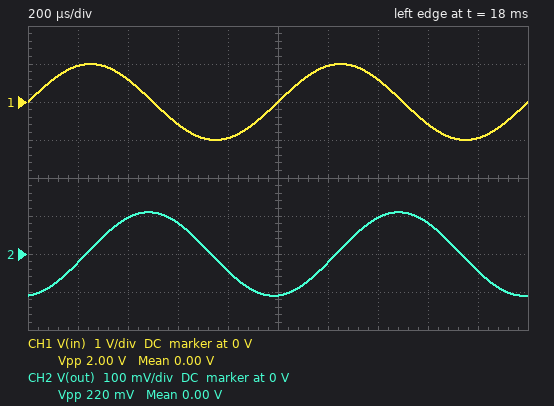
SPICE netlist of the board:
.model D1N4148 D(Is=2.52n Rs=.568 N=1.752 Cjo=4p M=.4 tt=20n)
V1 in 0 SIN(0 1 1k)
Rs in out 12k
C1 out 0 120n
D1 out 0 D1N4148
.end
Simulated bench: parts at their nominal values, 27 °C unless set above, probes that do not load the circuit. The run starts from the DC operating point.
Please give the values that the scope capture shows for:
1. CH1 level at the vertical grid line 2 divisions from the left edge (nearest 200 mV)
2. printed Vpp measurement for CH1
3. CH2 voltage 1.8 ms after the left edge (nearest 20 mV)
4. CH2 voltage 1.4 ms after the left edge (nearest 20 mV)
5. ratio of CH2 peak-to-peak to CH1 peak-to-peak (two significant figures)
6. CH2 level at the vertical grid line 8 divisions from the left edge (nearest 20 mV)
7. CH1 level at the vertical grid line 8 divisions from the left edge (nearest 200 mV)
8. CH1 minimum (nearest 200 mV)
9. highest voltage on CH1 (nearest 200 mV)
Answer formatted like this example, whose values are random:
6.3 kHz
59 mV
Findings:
600 mV
2.00 V
-40 mV
100 mV
0.11
80 mV
-600 mV
-1.0 V
1.0 V
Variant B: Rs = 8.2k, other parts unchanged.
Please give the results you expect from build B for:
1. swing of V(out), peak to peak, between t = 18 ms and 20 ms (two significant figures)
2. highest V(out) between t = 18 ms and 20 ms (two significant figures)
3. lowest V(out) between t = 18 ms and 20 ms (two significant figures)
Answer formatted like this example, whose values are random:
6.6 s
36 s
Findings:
320 mV
160 mV
-160 mV
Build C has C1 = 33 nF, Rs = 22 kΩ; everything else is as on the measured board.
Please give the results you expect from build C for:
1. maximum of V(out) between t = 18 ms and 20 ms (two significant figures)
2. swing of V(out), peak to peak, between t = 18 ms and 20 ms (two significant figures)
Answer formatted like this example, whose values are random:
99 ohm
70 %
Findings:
210 mV
430 mV
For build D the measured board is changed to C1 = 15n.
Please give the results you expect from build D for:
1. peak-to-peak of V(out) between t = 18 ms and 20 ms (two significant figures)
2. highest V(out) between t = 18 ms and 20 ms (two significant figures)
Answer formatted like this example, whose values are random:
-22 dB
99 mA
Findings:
1.1 V
440 mV
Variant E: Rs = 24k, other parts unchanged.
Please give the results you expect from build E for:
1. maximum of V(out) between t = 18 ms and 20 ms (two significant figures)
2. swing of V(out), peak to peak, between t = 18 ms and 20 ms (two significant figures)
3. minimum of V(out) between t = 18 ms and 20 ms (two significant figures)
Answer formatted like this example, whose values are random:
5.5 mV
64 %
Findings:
55 mV
110 mV
-55 mV
